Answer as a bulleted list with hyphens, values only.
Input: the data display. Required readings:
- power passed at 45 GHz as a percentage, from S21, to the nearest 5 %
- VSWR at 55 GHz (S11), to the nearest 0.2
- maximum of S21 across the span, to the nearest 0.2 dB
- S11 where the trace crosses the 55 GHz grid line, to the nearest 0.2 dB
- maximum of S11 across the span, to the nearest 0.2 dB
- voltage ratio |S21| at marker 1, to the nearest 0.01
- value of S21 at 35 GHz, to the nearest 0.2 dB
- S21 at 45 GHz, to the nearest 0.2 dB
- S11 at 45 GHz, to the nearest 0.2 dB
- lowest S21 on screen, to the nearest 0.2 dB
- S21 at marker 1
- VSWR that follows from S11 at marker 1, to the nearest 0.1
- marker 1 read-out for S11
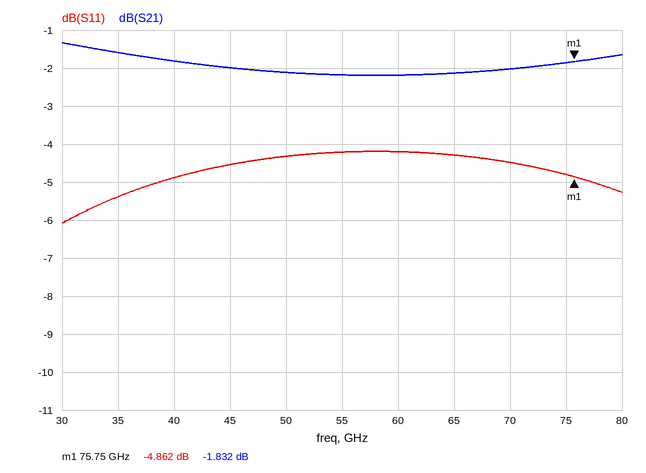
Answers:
- 65 %
- 4.2
- -1.4 dB
- -4.2 dB
- -4.2 dB
- 0.81
- -1.6 dB
- -2.0 dB
- -4.6 dB
- -2.2 dB
- -1.832 dB
- 3.7
- -4.862 dB
